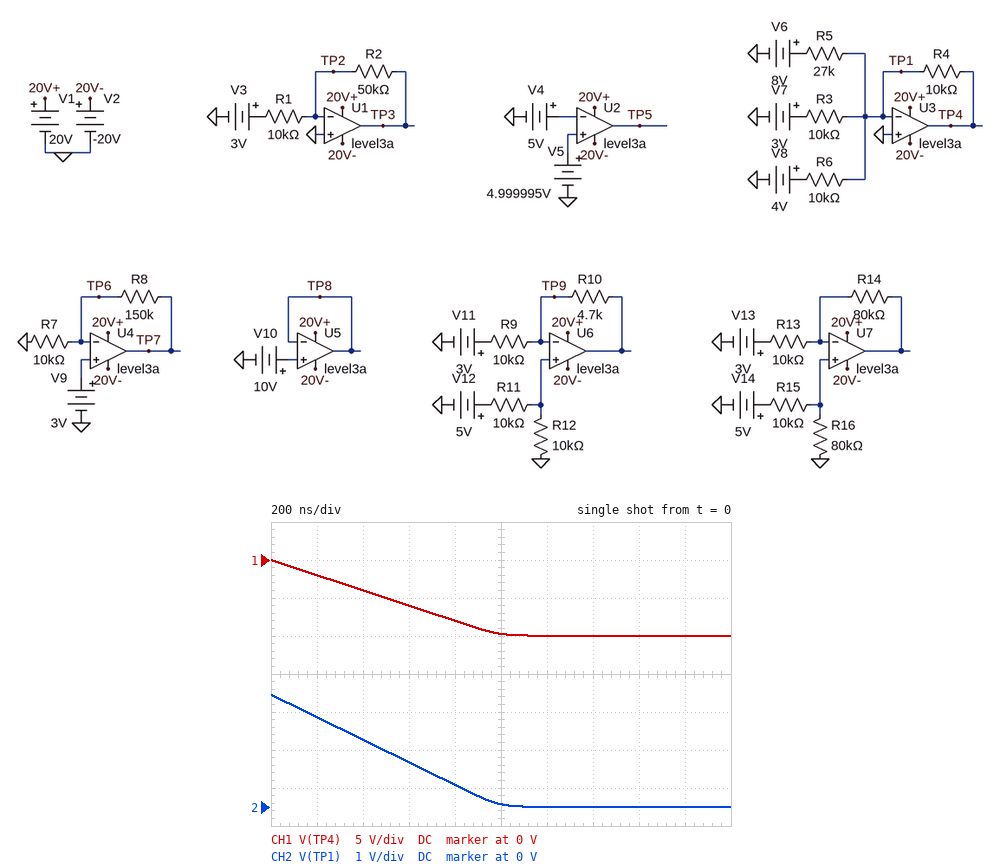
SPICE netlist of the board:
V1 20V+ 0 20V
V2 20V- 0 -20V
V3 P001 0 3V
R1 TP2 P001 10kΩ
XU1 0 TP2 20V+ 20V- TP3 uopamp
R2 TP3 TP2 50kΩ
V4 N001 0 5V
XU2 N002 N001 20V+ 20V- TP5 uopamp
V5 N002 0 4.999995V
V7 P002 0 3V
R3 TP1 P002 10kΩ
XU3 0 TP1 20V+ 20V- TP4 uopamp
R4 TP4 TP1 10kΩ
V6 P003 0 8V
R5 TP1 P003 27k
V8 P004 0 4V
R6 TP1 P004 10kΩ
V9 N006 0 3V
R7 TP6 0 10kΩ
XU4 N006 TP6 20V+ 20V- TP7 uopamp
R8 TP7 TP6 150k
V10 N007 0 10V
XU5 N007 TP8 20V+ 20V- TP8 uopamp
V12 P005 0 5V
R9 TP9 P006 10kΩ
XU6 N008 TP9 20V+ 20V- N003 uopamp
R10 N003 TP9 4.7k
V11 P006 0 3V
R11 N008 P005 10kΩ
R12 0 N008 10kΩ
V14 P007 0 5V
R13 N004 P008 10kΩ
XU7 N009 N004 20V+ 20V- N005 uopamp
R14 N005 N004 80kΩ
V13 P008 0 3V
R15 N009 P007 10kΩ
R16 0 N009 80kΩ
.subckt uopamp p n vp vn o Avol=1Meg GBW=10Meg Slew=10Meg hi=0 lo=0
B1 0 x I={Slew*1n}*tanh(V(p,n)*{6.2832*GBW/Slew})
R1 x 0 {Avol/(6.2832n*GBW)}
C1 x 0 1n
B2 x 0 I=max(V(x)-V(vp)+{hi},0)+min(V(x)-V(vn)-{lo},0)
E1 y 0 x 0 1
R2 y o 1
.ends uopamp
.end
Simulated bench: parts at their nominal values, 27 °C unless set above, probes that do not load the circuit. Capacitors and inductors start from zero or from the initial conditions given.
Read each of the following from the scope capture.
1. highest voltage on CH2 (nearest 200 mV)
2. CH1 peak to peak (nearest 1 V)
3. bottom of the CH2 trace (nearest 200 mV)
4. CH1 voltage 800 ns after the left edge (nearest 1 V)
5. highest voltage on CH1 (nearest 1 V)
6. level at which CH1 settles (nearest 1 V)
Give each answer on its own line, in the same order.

3.0 V
10 V
0 V
-8 V
0 V
-10 V
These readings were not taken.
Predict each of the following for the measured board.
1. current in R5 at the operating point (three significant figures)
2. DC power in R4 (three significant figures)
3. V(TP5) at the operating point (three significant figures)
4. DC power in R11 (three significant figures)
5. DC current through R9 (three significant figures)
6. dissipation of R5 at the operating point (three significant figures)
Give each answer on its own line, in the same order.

296 µA
9.93 mW
-5.00 V
625 µW
50.0 µA
2.37 mW
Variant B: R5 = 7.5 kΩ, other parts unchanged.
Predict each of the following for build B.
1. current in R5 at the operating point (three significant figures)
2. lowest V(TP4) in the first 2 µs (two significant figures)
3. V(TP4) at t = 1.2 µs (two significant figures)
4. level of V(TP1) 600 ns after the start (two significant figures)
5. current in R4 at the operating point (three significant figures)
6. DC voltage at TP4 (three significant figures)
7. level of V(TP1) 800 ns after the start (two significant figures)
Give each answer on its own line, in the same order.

1.07 mA
-18 V
-12 V
2.7 V
1.77 mA
-17.7 V
2.2 V
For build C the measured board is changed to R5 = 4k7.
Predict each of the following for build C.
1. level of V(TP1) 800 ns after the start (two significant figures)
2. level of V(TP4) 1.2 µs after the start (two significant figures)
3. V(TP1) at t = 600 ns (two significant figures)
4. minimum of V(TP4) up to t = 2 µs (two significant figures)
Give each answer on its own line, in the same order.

3.1 V
-12 V
3.5 V
-20 V
